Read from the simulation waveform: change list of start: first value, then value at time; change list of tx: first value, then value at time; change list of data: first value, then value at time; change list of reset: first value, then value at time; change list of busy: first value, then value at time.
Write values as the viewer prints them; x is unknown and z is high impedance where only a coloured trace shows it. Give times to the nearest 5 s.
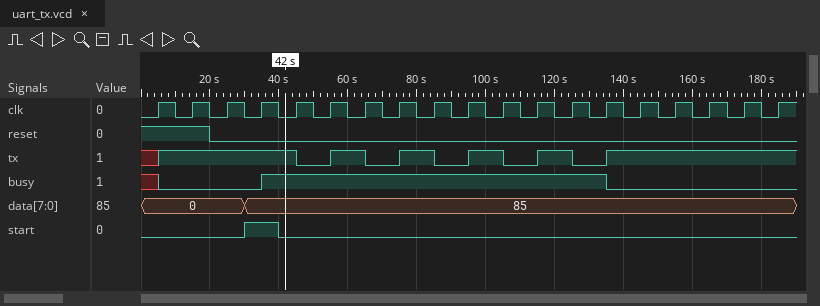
0, 1 at 30 s, 0 at 40 s
x, 1 at 5 s, 0 at 45 s, 1 at 55 s, 0 at 65 s, 1 at 75 s, 0 at 85 s, 1 at 95 s, 0 at 105 s, 1 at 115 s, 0 at 125 s, 1 at 135 s
0, 85 at 30 s
1, 0 at 20 s
x, 0 at 5 s, 1 at 35 s, 0 at 135 s
